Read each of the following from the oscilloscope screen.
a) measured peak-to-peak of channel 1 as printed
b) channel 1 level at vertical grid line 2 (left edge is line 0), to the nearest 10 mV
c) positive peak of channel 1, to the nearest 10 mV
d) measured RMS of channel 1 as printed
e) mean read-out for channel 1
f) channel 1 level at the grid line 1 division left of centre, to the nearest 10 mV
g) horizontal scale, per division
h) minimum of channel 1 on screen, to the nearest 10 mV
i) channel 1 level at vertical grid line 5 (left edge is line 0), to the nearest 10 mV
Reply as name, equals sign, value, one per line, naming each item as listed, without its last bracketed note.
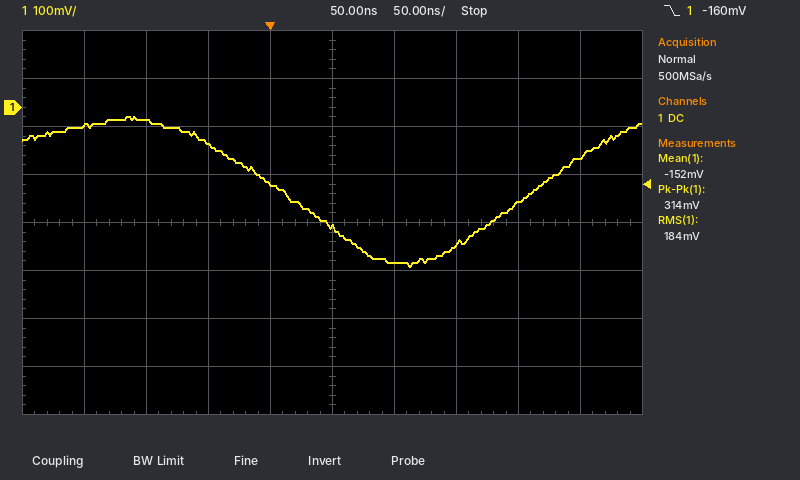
measured peak-to-peak of channel 1 as printed = 314 mV
channel 1 level at vertical grid line 2 (left edge is line 0), to the nearest 10 mV = -30 mV
positive peak of channel 1, to the nearest 10 mV = -20 mV
measured RMS of channel 1 as printed = 184 mV
mean read-out for channel 1 = -152 mV
channel 1 level at the grid line 1 division left of centre, to the nearest 10 mV = -160 mV
horizontal scale, per division = 50 ns
minimum of channel 1 on screen, to the nearest 10 mV = -330 mV
channel 1 level at vertical grid line 5 (left edge is line 0), to the nearest 10 mV = -250 mV
